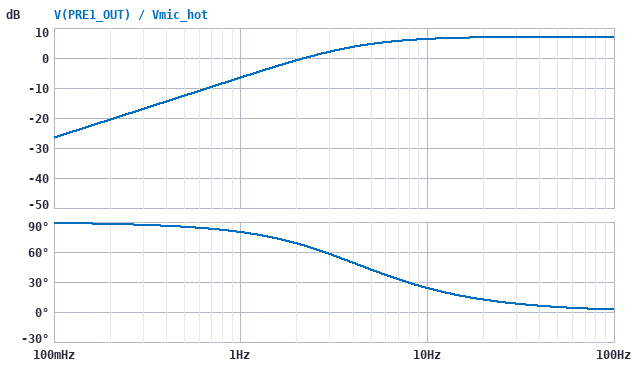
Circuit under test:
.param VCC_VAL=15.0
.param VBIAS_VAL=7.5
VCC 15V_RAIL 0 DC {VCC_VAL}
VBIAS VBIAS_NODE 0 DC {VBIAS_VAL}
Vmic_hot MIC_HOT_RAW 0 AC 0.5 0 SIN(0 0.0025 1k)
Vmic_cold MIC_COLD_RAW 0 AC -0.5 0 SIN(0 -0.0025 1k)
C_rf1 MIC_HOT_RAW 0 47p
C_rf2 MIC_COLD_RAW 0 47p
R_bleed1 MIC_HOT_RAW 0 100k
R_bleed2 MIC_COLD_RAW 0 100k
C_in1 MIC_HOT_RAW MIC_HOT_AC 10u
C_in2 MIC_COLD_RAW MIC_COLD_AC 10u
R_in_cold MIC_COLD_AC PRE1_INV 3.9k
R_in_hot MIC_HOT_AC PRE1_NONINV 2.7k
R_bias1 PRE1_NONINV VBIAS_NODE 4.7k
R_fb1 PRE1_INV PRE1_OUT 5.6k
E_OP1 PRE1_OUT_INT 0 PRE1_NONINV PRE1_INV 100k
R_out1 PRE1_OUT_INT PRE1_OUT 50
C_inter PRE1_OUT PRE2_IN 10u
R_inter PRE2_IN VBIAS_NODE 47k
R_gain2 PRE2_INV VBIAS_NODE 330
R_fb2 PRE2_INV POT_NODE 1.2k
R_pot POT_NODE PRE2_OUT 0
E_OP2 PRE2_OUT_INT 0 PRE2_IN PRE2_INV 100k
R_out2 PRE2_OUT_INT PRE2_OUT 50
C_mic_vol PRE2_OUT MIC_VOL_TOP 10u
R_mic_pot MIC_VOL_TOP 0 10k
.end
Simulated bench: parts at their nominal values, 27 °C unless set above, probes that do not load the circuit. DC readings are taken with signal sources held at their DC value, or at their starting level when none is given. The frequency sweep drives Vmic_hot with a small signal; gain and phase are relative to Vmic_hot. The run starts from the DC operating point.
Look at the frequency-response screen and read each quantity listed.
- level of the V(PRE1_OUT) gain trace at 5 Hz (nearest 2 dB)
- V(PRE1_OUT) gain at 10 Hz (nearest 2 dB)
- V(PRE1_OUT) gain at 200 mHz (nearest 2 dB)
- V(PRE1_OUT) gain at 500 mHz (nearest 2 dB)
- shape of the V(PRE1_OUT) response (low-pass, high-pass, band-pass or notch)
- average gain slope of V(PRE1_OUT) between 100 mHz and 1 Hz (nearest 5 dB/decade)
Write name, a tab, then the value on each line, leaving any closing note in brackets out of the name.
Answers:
level of the V(PRE1_OUT) gain trace at 5 Hz	4 dB
V(PRE1_OUT) gain at 10 Hz	6 dB
V(PRE1_OUT) gain at 200 mHz	-20 dB
V(PRE1_OUT) gain at 500 mHz	-12 dB
shape of the V(PRE1_OUT) response	high-pass
average gain slope of V(PRE1_OUT) between 100 mHz and 1 Hz	20 dB/decade
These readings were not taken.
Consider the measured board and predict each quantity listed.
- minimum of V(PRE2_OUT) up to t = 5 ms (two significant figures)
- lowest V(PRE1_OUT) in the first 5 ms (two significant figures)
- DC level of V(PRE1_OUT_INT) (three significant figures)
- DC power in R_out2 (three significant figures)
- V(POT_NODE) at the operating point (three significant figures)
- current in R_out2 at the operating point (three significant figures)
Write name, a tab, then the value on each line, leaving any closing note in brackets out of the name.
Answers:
minimum of V(PRE2_OUT) up to t = 5 ms	7.5 V
lowest V(PRE1_OUT) in the first 5 ms	7.5 V
DC level of V(PRE1_OUT_INT)	7.50 V
DC power in R_out2	4.65 µW
V(POT_NODE) at the operating point	7.50 V
current in R_out2 at the operating point	305 µA
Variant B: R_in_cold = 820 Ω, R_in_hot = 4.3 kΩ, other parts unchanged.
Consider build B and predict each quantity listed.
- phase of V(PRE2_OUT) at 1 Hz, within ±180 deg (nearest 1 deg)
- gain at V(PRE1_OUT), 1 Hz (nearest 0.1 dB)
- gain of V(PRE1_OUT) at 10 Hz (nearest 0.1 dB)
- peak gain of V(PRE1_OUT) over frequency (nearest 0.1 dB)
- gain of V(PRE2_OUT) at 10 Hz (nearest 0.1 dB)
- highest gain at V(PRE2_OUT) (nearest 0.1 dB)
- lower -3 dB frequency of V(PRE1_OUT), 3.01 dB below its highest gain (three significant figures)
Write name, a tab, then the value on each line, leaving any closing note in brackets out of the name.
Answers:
phase of V(PRE2_OUT) at 1 Hz, within ±180 deg	101 deg
gain at V(PRE1_OUT), 1 Hz	-6.9 dB
gain of V(PRE1_OUT) at 10 Hz	10.8 dB
peak gain of V(PRE1_OUT) over frequency	17.5 dB
gain of V(PRE2_OUT) at 10 Hz	24.1 dB
highest gain at V(PRE2_OUT)	30.8 dB
lower -3 dB frequency of V(PRE1_OUT), 3.01 dB below its highest gain	19.3 Hz
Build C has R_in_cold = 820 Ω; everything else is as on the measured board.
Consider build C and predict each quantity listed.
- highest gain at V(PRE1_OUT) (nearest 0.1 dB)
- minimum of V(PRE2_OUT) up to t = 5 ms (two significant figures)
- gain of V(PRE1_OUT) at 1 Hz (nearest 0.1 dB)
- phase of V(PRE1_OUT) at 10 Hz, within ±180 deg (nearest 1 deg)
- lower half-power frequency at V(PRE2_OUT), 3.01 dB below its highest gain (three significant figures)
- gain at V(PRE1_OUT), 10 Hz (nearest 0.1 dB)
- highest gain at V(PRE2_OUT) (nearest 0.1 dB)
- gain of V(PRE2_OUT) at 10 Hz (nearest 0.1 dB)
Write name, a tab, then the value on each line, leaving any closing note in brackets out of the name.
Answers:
highest gain at V(PRE1_OUT)	18.5 dB
minimum of V(PRE2_OUT) up to t = 5 ms	7.4 V
gain of V(PRE1_OUT) at 1 Hz	-6.7 dB
phase of V(PRE1_OUT) at 10 Hz, within ±180 deg	62 deg
lower half-power frequency at V(PRE2_OUT), 3.01 dB below its highest gain	19.4 Hz
gain at V(PRE1_OUT), 10 Hz	11.7 dB
highest gain at V(PRE2_OUT)	31.8 dB
gain of V(PRE2_OUT) at 10 Hz	25.0 dB
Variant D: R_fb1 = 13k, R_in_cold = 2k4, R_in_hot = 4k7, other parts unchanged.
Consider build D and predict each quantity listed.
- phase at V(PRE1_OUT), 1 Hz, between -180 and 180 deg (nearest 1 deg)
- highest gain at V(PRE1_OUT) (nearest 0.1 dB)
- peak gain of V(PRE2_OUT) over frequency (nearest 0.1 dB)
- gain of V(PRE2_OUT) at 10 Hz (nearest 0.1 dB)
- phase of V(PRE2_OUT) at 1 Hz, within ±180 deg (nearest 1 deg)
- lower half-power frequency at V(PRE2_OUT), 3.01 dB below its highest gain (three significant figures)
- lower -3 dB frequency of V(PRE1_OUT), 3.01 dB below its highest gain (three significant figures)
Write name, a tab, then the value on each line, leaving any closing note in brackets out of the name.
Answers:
phase at V(PRE1_OUT), 1 Hz, between -180 and 180 deg	88 deg
highest gain at V(PRE1_OUT)	15.4 dB
peak gain of V(PRE2_OUT) over frequency	28.8 dB
gain of V(PRE2_OUT) at 10 Hz	27.1 dB
phase of V(PRE2_OUT) at 1 Hz, within ±180 deg	106 deg
lower half-power frequency at V(PRE2_OUT), 3.01 dB below its highest gain	6.80 Hz
lower -3 dB frequency of V(PRE1_OUT), 3.01 dB below its highest gain	6.78 Hz
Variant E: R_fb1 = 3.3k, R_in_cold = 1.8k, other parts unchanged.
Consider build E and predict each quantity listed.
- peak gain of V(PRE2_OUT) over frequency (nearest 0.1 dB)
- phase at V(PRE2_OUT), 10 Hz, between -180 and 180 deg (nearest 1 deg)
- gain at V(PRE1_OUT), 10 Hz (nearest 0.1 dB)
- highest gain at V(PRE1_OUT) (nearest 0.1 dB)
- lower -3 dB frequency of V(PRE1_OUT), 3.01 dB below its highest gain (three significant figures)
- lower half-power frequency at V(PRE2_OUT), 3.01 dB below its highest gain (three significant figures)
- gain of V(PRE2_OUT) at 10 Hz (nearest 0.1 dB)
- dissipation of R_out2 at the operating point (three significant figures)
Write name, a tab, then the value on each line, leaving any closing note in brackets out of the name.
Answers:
peak gain of V(PRE2_OUT) over frequency	22.0 dB
phase at V(PRE2_OUT), 10 Hz, between -180 and 180 deg	40 deg
gain at V(PRE1_OUT), 10 Hz	6.3 dB
highest gain at V(PRE1_OUT)	8.7 dB
lower -3 dB frequency of V(PRE1_OUT), 3.01 dB below its highest gain	8.50 Hz
lower half-power frequency at V(PRE2_OUT), 3.01 dB below its highest gain	8.51 Hz
gain of V(PRE2_OUT) at 10 Hz	19.6 dB
dissipation of R_out2 at the operating point	4.65 µW
